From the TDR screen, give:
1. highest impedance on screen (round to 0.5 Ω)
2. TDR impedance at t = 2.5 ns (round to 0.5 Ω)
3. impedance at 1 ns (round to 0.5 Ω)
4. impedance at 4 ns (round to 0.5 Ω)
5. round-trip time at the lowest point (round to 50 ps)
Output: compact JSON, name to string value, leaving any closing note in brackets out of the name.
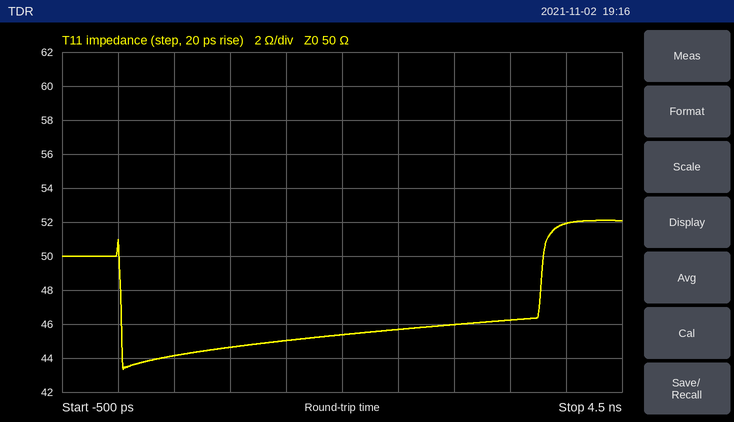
{"highest impedance on screen": "52.0 Ω", "TDR impedance at t = 2.5 ns": "45.5 Ω", "impedance at 1 ns": "44.5 Ω", "impedance at 4 ns": "52.0 Ω", "round-trip time at the lowest point": "50 ps"}
